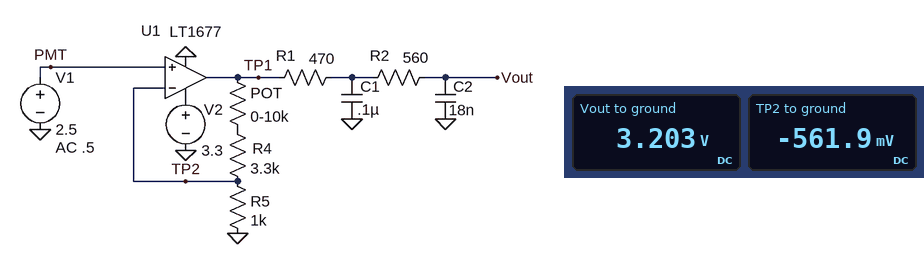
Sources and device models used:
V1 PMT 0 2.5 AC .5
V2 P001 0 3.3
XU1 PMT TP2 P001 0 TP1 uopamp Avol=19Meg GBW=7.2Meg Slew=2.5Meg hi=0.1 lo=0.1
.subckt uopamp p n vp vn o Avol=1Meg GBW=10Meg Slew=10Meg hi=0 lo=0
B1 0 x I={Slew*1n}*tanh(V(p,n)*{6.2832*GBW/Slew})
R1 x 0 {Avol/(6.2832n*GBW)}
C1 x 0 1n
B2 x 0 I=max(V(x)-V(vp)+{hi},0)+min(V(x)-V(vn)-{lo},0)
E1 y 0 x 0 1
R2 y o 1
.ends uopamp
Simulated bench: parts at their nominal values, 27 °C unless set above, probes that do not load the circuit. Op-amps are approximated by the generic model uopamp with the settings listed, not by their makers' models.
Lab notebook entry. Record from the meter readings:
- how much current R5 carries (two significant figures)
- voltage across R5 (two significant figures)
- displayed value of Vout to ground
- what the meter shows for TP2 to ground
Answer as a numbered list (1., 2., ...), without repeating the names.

1. 560 µA
2. 560 mV
3. 3.203 V
4. -561.9 mV
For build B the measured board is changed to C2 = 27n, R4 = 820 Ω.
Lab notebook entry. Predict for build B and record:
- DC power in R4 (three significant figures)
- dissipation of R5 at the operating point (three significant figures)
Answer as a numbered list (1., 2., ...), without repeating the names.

1. 126 µW
2. 153 µW
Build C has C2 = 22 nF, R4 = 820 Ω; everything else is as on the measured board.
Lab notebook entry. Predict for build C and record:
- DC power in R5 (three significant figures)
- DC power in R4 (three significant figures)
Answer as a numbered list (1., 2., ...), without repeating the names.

1. 153 µW
2. 126 µW
